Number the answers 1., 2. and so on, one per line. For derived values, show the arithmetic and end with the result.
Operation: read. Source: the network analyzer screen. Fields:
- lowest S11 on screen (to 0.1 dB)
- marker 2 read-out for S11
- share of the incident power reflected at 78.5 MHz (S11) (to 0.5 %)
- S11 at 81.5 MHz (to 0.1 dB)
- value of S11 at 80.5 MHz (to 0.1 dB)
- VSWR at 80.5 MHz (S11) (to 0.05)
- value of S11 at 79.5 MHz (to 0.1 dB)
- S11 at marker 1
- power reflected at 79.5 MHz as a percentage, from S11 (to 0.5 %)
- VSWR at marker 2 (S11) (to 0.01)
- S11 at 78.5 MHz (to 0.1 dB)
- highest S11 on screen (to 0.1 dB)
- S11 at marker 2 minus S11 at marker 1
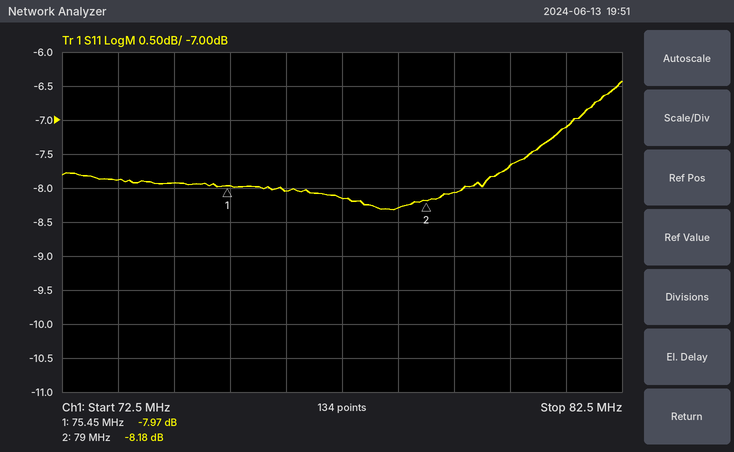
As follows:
1. -8.3 dB
2. -8.18 dB
3. 10^(-8.3/10) ≈ 14.8 %, so 15.0 % to the nearest 0.5 %
4. -7.1 dB
5. -7.7 dB
6. |Γ| = 10^(-7.7/20) = 0.4121; VSWR = (1 + 0.4121)/(1 − 0.4121) ≈ 2.40
7. -8.1 dB
8. -7.97 dB
9. 10^(-8.1/10) ≈ 15.5 %
10. (1 + 0.3899)/(1 − 0.3899) ≈ 2.28
11. -8.3 dB
12. -6.4 dB
13. -8.18 − (-7.97) = -0.21 dB
